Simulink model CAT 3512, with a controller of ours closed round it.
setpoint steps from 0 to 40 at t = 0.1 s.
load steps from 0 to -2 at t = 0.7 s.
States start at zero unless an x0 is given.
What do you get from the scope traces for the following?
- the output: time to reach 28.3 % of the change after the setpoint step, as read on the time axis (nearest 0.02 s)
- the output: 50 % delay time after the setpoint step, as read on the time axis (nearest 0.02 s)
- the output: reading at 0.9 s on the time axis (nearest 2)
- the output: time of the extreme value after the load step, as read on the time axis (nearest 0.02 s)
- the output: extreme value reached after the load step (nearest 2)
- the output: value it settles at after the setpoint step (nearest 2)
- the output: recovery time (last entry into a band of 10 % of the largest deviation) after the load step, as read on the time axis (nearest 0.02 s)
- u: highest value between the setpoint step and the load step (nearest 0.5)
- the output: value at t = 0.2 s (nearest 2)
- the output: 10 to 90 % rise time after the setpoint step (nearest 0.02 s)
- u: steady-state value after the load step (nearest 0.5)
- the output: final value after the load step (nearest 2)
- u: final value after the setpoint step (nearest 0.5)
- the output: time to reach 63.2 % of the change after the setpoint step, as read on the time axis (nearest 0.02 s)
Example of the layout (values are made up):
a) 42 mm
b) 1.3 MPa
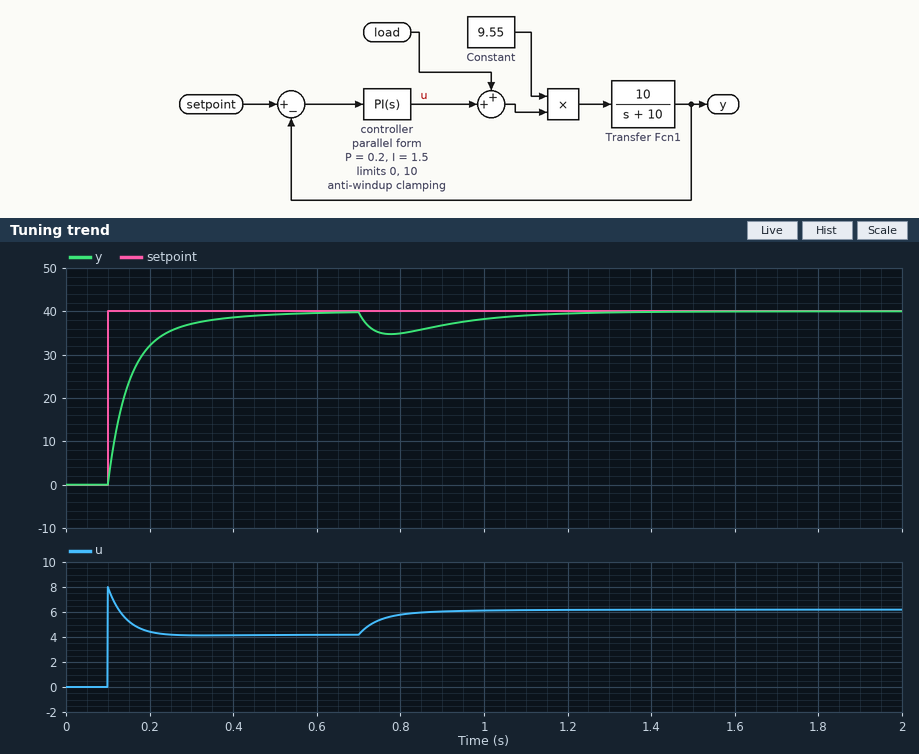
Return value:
a) 0.12 s
b) 0.14 s
c) 36
d) 0.78 s
e) 34
f) 40
g) 1.20 s
h) 8.0
i) 32
j) 0.16 s
k) 6.0
l) 40
m) 4.0
n) 0.16 s
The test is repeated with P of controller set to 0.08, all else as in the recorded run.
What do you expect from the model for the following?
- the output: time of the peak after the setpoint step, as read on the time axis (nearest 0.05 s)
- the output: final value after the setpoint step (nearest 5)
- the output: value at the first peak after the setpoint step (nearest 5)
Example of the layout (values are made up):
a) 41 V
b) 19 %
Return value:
a) 0.40 s
b) 40
c) 40
